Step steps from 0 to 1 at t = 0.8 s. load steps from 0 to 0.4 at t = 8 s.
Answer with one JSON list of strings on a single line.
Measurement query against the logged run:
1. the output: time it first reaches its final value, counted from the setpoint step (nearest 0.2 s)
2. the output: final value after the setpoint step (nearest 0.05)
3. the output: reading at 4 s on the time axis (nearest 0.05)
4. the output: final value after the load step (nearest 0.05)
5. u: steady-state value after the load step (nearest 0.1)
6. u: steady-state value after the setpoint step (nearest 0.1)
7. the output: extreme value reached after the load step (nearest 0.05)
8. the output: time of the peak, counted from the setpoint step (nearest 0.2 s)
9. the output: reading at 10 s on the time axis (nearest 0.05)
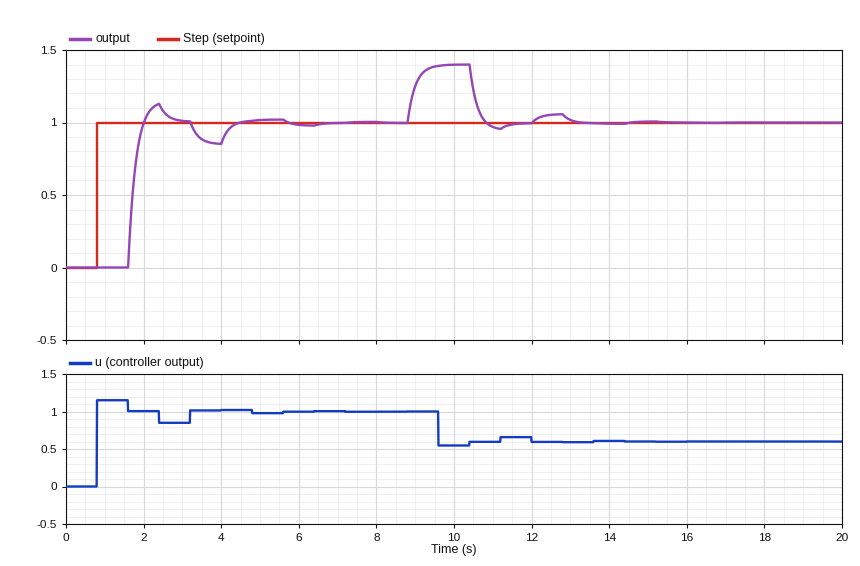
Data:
["1.2 s", "1.00", "0.85", "1.00", "0.6", "1.0", "1.40", "1.6 s", "1.40"]
